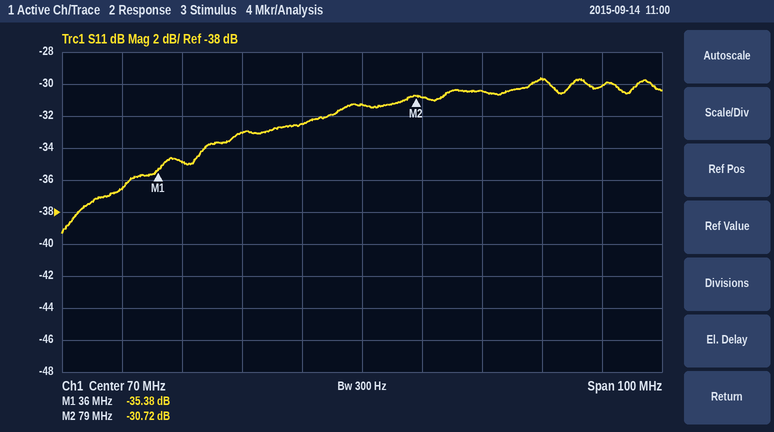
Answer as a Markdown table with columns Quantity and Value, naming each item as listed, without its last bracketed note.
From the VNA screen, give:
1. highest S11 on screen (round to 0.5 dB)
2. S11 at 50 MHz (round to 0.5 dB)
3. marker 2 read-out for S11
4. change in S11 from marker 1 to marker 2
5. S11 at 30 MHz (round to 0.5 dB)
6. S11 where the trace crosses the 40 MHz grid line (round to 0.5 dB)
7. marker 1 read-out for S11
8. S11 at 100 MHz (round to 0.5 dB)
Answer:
| Quantity | Value |
|---|---|
| highest S11 on screen | -29.5 dB |
| S11 at 50 MHz | -33.0 dB |
| marker 2 read-out for S11 | -30.72 dB |
| change in S11 from marker 1 to marker 2 | 4.66 dB |
| S11 at 30 MHz | -36.5 dB |
| S11 where the trace crosses the 40 MHz grid line | -35.0 dB |
| marker 1 read-out for S11 | -35.38 dB |
| S11 at 100 MHz | -29.5 dB |
